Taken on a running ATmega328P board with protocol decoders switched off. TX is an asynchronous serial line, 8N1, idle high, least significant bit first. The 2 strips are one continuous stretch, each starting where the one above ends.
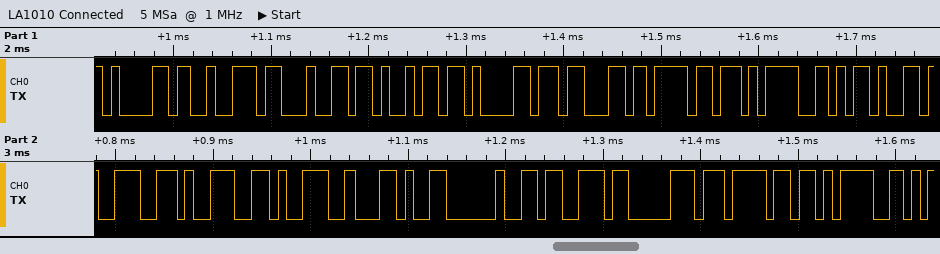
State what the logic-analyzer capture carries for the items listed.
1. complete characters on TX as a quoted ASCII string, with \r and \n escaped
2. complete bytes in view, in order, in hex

"ardiaco=-999, spo="
0x61 0x72 0x64 0x69 0x61 0x63 0x6F 0x3D 0x2D 0x39 0x39 0x39 0x2C 0x20 0x73 0x70 0x6F 0x3D
